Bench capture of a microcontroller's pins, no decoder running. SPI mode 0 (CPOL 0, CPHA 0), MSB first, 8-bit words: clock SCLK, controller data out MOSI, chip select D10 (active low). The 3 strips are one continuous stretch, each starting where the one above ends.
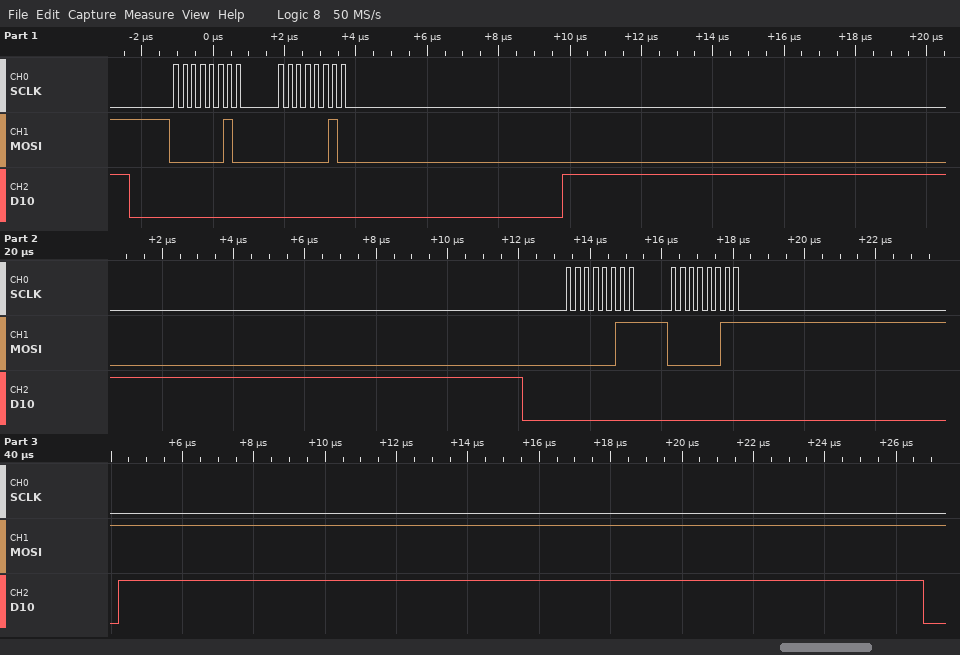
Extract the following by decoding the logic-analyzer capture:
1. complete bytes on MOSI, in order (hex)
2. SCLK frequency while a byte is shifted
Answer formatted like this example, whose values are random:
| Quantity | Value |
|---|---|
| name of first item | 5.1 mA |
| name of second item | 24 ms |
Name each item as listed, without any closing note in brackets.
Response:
| Quantity | Value |
|---|---|
| complete bytes on MOSI, in order | 02 02 03 03 |
| SCLK frequency while a byte is shifted | 4 MHz |
